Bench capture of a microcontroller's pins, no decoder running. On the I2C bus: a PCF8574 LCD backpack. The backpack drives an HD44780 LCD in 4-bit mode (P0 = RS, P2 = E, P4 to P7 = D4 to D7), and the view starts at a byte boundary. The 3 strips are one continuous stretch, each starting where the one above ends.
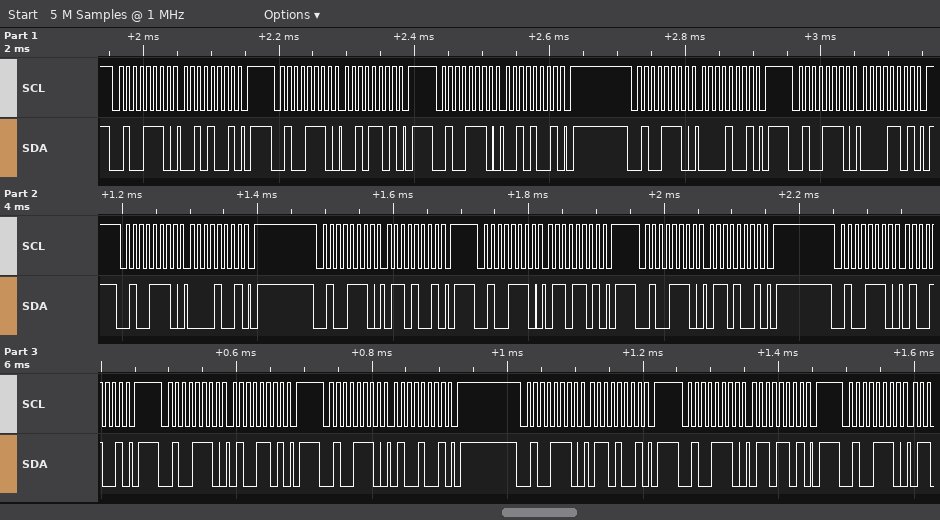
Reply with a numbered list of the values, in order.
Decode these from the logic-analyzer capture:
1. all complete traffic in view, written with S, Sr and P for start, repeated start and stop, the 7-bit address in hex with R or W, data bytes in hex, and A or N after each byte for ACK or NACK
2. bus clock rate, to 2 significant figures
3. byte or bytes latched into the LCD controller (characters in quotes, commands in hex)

1. S 27W A 29 A P S 27W A 2D A P S 27W A 29 A P S 27W A 09 A P S 27W A 0D A P S 27W A 09 A P S 27W A 69 A P S 27W A 6D A P S 27W A 69 A P S 27W A 49 A P S 27W A 4D A P S 27W A 49 A P S 27W A 69 A P S 27W A 6D A P S 27W A
2. 100 kHz
3. ' ' 'd'
